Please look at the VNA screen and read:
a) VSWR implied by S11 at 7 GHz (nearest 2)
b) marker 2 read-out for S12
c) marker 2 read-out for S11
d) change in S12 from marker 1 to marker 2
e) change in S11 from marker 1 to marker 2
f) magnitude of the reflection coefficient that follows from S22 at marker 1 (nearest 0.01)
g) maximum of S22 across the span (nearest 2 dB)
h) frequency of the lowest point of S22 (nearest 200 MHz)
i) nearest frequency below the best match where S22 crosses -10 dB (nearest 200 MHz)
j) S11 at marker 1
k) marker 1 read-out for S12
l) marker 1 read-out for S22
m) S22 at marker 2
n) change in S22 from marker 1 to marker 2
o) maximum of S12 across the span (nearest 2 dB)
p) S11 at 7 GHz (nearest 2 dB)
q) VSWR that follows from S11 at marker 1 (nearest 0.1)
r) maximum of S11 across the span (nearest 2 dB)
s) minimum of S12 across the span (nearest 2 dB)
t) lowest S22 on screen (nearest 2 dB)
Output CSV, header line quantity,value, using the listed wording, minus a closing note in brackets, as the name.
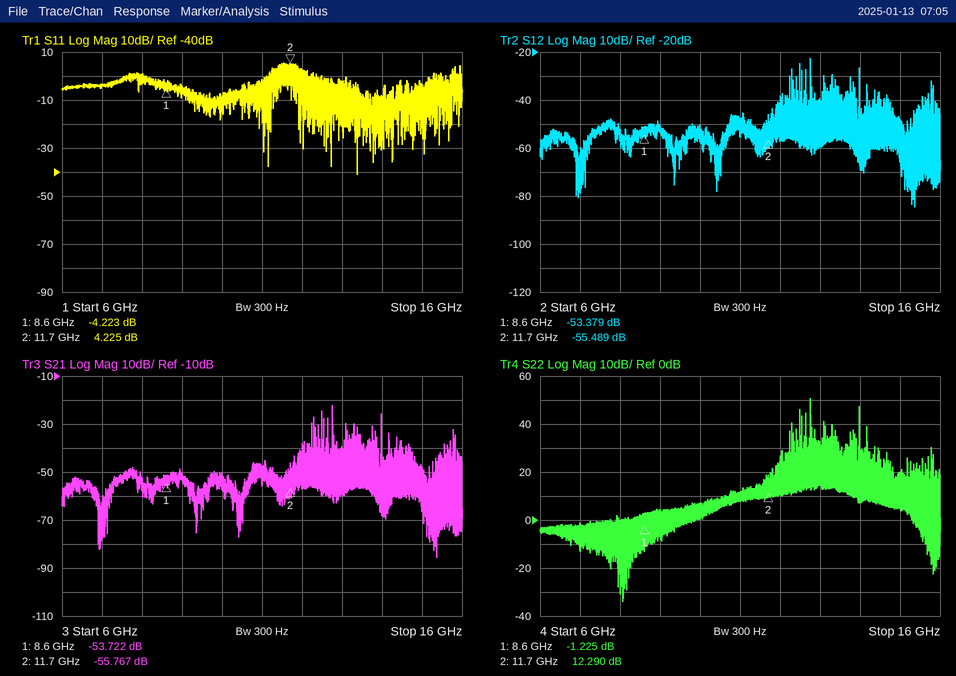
quantity,value
VSWR implied by S11 at 7 GHz,4
marker 2 read-out for S12,-55.489 dB
marker 2 read-out for S11,4.225 dB
change in S12 from marker 1 to marker 2,-2.110 dB
change in S11 from marker 1 to marker 2,8.448 dB
magnitude of the reflection coefficient that follows from S22 at marker 1,0.87
maximum of S22 across the span,50 dB
frequency of the lowest point of S22,8.0 GHz
nearest frequency below the best match where S22 crosses -10 dB,8.0 GHz
S11 at marker 1,-4.223 dB
marker 1 read-out for S12,-53.379 dB
marker 1 read-out for S22,-1.225 dB
S22 at marker 2,12.290 dB
change in S22 from marker 1 to marker 2,13.515 dB
maximum of S12 across the span,-22 dB
S11 at 7 GHz,-4 dB
VSWR that follows from S11 at marker 1,4.2
maximum of S11 across the span,6 dB
minimum of S12 across the span,-84 dB
lowest S22 on screen,-34 dB
